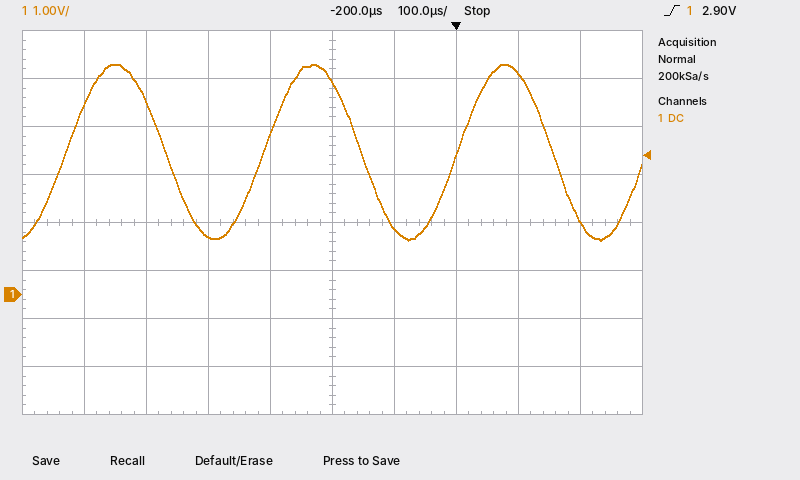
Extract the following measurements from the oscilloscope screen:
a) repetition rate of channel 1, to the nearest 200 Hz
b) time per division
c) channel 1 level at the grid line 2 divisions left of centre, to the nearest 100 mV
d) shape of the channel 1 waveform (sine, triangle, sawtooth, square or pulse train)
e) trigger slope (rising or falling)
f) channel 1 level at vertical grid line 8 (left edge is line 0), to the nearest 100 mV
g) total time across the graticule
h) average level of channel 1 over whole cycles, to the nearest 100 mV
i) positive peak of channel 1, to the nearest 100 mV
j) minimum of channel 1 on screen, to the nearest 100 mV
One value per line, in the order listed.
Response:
3.2 kHz
100 µs
1.2 V
sine
rising
4.6 V
1 ms
3.0 V
4.8 V
1.1 V
